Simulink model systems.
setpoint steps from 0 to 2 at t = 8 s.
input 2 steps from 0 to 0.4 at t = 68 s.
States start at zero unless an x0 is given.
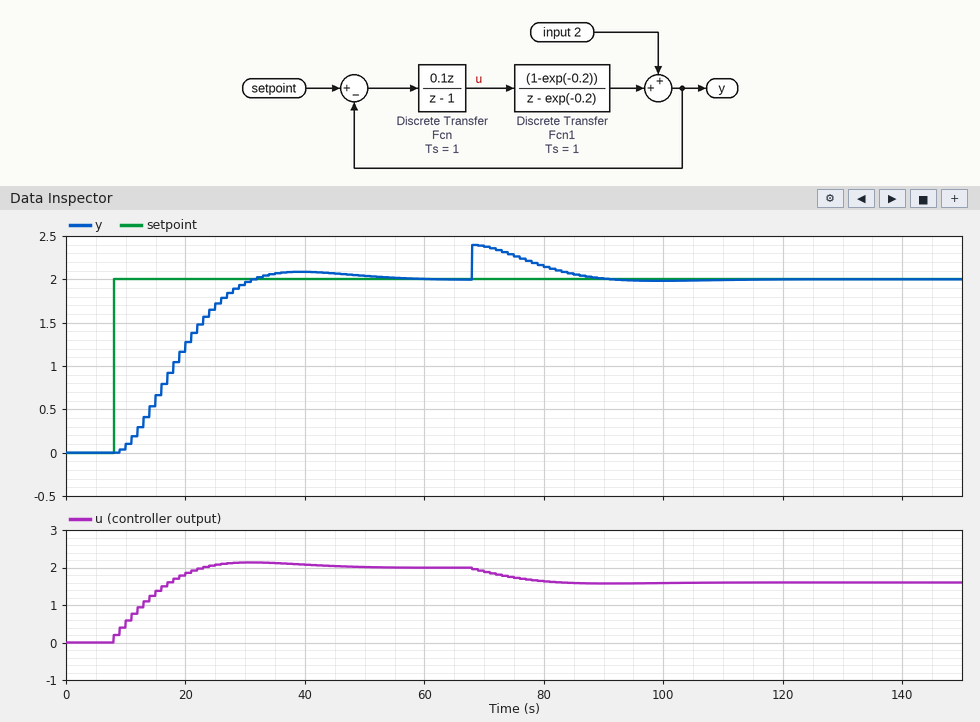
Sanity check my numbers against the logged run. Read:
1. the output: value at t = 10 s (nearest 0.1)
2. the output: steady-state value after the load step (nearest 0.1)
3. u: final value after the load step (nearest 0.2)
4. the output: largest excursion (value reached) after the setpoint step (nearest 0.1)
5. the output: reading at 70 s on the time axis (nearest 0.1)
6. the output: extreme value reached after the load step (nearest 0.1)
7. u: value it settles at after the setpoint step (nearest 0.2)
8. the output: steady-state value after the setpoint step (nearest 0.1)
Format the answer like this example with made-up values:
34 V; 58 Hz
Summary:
0.1; 2.0; 1.6; 2.1; 2.4; 2.4; 2.0; 2.0
